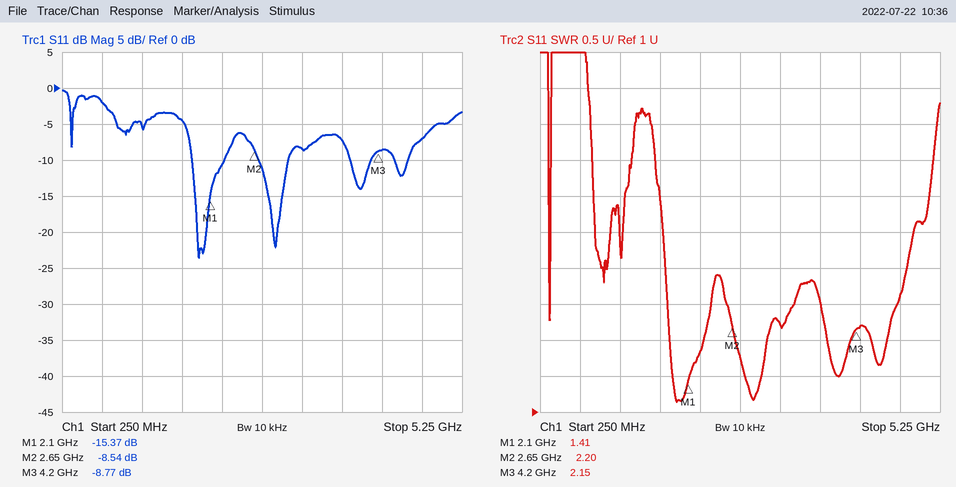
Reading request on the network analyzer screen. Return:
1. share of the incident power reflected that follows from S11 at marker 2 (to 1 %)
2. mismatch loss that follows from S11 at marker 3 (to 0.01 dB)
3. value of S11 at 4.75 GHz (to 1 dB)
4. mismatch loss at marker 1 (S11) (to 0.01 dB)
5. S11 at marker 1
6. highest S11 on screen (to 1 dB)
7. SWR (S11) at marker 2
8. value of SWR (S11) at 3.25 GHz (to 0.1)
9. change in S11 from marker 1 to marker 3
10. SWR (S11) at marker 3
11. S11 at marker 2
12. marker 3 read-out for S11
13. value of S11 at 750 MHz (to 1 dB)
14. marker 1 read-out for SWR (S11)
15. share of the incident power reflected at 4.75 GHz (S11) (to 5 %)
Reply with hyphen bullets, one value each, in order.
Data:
- 14 %
- 0.62 dB
- -7 dB
- 0.13 dB
- -15.37 dB
- 0 dB
- 2.20
- 2.2
- 6.60 dB
- 2.15
- -8.54 dB
- -8.77 dB
- -2 dB
- 1.41
- 20 %
